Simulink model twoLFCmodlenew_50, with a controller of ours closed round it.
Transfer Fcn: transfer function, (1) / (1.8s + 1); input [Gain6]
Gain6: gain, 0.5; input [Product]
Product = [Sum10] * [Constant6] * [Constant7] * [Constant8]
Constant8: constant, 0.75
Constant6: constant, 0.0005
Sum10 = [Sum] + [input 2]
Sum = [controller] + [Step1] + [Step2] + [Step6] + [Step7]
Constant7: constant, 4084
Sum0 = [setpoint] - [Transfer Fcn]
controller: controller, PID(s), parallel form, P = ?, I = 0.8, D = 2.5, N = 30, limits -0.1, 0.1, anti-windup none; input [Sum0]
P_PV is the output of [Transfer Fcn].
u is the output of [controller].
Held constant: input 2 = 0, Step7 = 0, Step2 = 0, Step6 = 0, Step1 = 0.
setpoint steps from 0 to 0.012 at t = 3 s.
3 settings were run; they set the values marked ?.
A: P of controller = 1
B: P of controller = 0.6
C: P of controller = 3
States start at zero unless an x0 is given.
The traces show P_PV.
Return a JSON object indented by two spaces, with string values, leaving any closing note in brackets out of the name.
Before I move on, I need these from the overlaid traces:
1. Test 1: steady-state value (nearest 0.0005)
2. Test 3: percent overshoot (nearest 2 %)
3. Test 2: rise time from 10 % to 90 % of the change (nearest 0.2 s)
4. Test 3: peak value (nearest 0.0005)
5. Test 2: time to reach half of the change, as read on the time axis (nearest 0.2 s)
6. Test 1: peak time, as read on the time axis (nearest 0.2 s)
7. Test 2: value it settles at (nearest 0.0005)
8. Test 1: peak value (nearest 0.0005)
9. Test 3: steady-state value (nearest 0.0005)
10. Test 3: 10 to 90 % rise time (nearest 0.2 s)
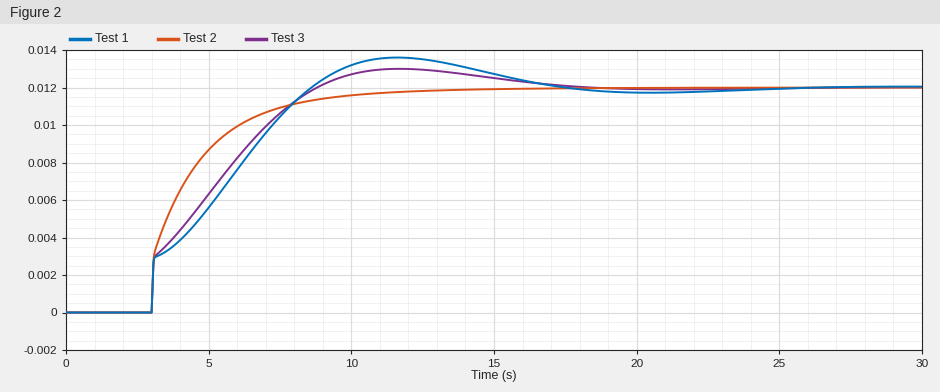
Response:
{
  "Test 1: steady-state value": "0.0120",
  "Test 3: percent overshoot": "8 %",
  "Test 2: rise time from 10 % to 90 % of the change": "4.2 s",
  "Test 3: peak value": "0.0130",
  "Test 2: time to reach half of the change, as read on the time axis": "3.8 s",
  "Test 1: peak time, as read on the time axis": "11.6 s",
  "Test 2: value it settles at": "0.0120",
  "Test 1: peak value": "0.0135",
  "Test 3: steady-state value": "0.0120",
  "Test 3: 10 to 90 % rise time": "4.6 s"
}
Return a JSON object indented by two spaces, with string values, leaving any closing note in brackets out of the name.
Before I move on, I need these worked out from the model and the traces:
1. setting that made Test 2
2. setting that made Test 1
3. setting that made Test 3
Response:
{
  "setting that made Test 2": "C",
  "setting that made Test 1": "B",
  "setting that made Test 3": "A"
}
